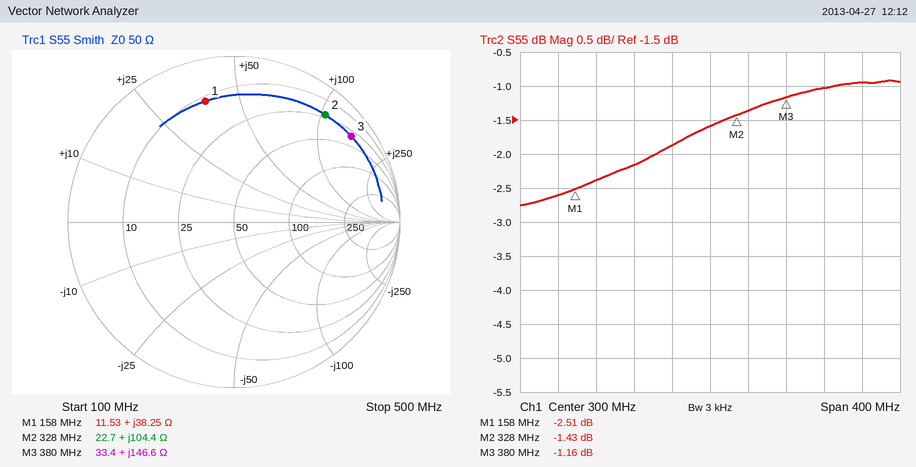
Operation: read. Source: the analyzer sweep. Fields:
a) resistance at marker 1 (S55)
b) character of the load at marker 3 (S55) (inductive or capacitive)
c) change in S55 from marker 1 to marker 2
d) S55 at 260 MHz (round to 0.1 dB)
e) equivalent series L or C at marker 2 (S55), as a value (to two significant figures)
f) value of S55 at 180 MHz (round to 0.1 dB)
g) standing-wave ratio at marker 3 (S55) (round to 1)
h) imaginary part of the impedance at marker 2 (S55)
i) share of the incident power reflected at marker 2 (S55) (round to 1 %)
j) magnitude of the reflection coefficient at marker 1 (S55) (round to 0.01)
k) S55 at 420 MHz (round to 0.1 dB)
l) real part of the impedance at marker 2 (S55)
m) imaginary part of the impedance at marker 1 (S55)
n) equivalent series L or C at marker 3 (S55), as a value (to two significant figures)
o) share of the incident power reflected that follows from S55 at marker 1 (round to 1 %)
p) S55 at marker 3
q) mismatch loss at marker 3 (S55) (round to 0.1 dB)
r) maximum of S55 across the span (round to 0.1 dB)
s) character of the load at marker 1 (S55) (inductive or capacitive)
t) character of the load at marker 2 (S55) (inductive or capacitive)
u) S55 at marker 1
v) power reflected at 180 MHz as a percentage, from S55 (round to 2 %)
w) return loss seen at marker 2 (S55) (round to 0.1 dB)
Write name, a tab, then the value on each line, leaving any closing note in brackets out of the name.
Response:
resistance at marker 1	11.53 Ω
character of the load at marker 3 (S55)	inductive
change in S55 from marker 1 to marker 2	1.08 dB
S55 at 260 MHz	-1.9 dB
equivalent series L or C at marker 2 (S55), as a value	51 nH
value of S55 at 180 MHz	-2.4 dB
standing-wave ratio at marker 3 (S55)	15
imaginary part of the impedance at marker 2	+104.4 Ω
share of the incident power reflected at marker 2 (S55)	72 %
magnitude of the reflection coefficient at marker 1 (S55)	0.75
S55 at 420 MHz	-1.0 dB
real part of the impedance at marker 2	22.7 Ω
imaginary part of the impedance at marker 1	+38.25 Ω
equivalent series L or C at marker 3 (S55), as a value	61 nH
share of the incident power reflected that follows from S55 at marker 1	56 %
S55 at marker 3	-1.16 dB
mismatch loss at marker 3 (S55)	6.3 dB
maximum of S55 across the span	-0.9 dB
character of the load at marker 1 (S55)	inductive
character of the load at marker 2 (S55)	inductive
S55 at marker 1	-2.51 dB
power reflected at 180 MHz as a percentage, from S55	58 %
return loss seen at marker 2 (S55)	1.4 dB
